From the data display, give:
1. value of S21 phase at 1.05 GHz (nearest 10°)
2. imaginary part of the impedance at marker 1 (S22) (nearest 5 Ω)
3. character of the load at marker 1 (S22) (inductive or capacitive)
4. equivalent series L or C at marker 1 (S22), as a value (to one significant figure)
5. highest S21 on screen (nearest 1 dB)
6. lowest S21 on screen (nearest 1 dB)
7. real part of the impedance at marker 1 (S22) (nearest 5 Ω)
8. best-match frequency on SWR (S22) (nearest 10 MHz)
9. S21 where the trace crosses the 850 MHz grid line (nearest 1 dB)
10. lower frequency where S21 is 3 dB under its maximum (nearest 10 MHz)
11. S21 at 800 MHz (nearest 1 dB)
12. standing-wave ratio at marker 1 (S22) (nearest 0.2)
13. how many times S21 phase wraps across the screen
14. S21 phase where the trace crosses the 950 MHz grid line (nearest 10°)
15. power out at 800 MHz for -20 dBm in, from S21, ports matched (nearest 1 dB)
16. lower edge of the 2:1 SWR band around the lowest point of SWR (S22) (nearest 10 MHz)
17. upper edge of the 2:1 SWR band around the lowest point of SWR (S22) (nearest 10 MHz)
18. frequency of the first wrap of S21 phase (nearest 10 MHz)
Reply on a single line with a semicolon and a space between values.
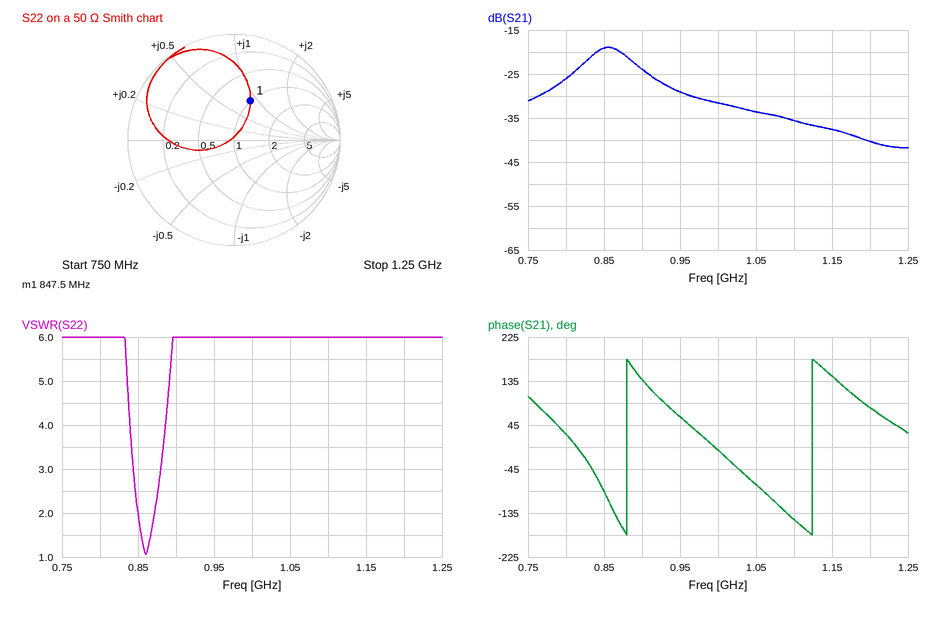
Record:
-80°; +45 Ω; inductive; 8 nH; -19 dB; -42 dB; 50 Ω; 860 MHz; -19 dB; 830 MHz; -26 dB; 2.4; 2; 60°; -46 dBm; 850 MHz; 870 MHz; 880 MHz
